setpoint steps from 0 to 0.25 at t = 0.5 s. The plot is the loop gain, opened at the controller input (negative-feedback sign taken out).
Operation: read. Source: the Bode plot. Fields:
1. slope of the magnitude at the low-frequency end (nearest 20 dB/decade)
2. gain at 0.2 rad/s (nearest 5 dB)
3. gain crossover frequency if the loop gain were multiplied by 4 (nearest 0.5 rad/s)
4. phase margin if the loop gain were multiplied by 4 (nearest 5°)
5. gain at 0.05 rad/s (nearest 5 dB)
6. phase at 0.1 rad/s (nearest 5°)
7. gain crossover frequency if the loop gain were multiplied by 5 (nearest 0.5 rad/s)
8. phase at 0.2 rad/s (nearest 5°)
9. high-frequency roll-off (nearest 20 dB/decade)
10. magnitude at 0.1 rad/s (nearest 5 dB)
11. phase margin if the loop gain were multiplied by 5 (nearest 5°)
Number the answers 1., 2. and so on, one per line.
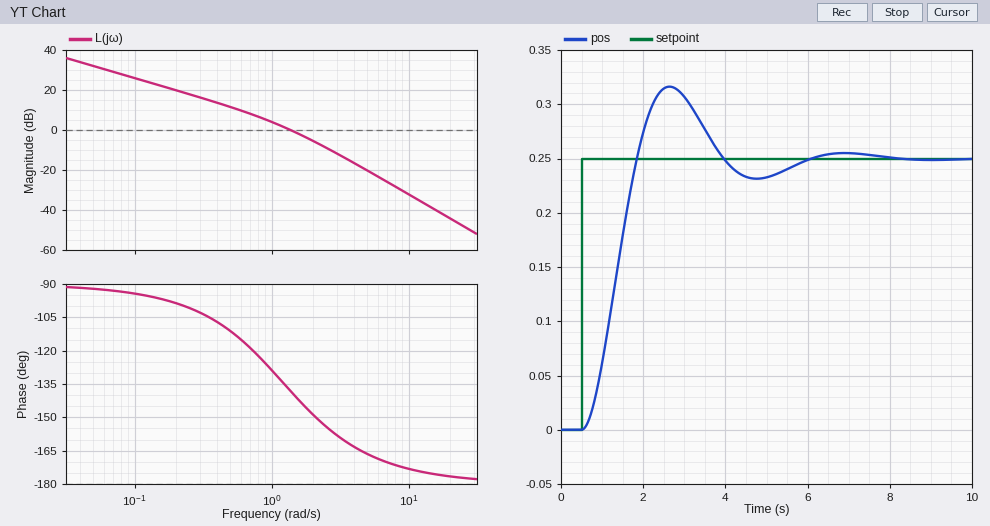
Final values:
1. -20 dB/decade
2. 20 dB
3. 3.0 rad/s
4. 20°
5. 30 dB
6. -95°
7. 3.5 rad/s
8. -100°
9. -40 dB/decade
10. 25 dB
11. 20°
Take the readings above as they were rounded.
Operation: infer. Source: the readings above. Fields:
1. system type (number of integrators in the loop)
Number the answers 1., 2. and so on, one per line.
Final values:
1. 1
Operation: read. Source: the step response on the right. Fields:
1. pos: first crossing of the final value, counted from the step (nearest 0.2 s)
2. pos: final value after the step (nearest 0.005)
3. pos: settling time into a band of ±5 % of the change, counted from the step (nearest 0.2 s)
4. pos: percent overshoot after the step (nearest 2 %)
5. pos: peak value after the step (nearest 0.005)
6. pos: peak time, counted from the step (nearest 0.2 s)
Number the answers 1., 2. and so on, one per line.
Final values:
1. 1.4 s
2. 0.250
3. 4.8 s
4. 26 %
5. 0.315
6. 2.2 s
